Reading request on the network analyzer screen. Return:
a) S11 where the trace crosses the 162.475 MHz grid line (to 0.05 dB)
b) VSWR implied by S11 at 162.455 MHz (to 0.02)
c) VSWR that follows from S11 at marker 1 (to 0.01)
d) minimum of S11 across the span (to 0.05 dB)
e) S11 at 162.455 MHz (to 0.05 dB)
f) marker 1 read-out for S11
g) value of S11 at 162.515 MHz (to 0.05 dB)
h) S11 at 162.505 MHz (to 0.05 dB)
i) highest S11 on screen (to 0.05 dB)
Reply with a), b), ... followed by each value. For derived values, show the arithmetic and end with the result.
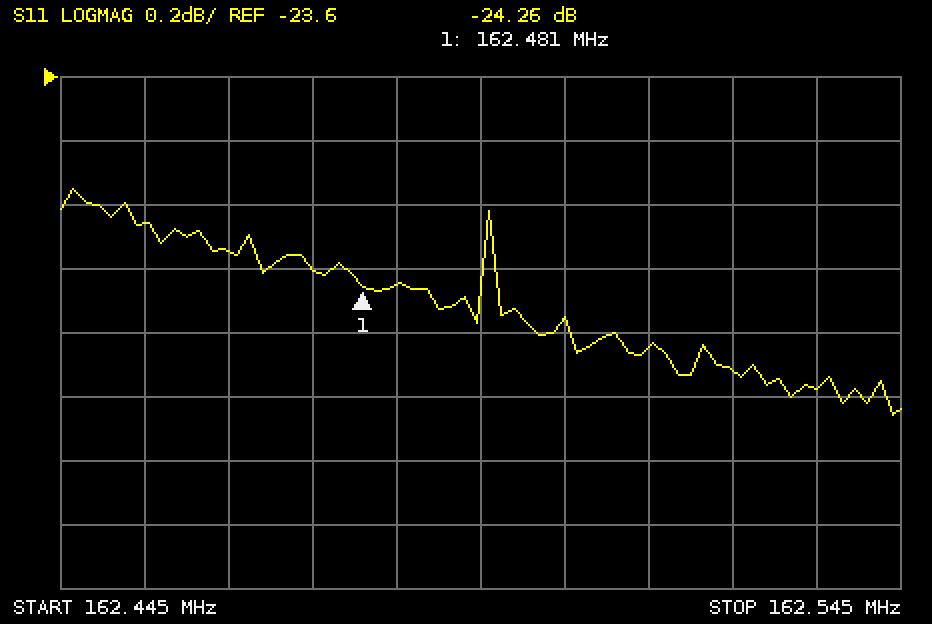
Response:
a) -24.20 dB
b) |Γ| = 10^(-24.05/20) = 0.0627; VSWR = (1 + 0.0627)/(1 − 0.0627) ≈ 1.13, so 1.14 to the nearest 0.02
c) (1 + 0.0612)/(1 − 0.0612) ≈ 1.13
d) -24.65 dB
e) -24.05 dB
f) -24.26 dB
g) -24.45 dB
h) -24.35 dB
i) -23.95 dB
